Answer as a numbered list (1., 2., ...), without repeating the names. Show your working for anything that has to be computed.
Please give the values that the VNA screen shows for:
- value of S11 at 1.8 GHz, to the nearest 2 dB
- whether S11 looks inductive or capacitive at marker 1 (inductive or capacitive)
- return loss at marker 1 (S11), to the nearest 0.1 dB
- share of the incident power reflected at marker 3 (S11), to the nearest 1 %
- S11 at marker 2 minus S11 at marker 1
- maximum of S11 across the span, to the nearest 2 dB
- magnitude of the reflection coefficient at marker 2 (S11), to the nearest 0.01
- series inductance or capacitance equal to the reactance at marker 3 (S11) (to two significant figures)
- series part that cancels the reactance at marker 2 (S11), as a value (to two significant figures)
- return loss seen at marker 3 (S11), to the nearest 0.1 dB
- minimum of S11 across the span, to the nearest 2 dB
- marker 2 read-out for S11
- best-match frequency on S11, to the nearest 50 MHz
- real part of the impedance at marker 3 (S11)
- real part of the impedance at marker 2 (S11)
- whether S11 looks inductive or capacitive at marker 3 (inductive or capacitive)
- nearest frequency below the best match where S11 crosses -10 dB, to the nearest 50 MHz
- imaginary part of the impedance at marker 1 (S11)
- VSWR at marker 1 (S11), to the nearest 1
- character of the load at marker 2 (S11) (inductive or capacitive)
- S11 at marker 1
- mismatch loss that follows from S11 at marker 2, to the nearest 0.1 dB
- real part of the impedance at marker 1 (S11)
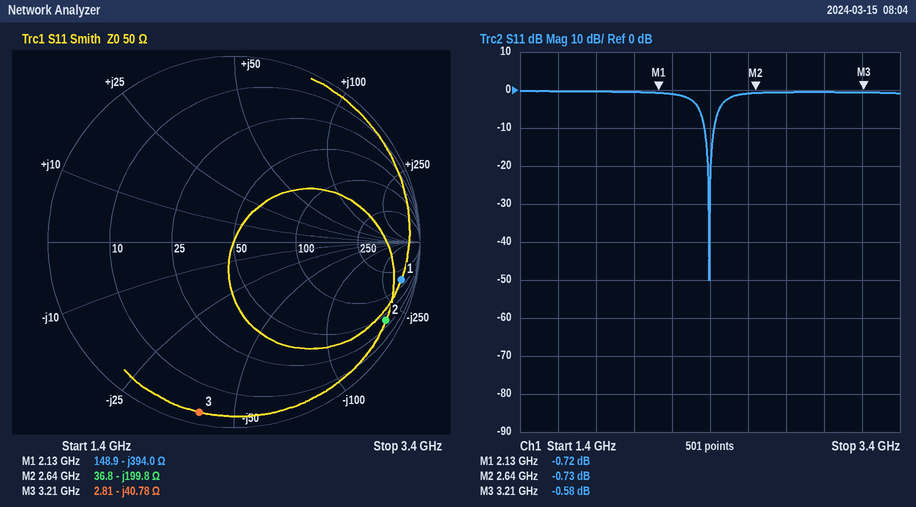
1. 0 dB
2. capacitive
3. 0.7 dB
4. 10^(-0.58/10) ≈ 87 %
5. -0.73 − (-0.72) = -0.01 dB
6. 0 dB
7. 0.92
8. C = 1/(2π × 3.21 GHz × 40.78 Ω) ≈ 1.2 pF
9. L = 199.8 Ω/(2π × 2.64 GHz) ≈ 12 nH
10. 0.6 dB
11. -50 dB
12. -0.73 dB
13. 2.40 GHz
14. 2.81 Ω
15. 36.8 Ω
16. capacitive
17. 2.35 GHz
18. -394.0 Ω
19. (1 + 0.9204)/(1 − 0.9204) ≈ 24
20. capacitive
21. -0.72 dB
22. −10 log10(1 − 10^(-0.73/10)) ≈ 8.1 dB
23. 148.9 Ω
